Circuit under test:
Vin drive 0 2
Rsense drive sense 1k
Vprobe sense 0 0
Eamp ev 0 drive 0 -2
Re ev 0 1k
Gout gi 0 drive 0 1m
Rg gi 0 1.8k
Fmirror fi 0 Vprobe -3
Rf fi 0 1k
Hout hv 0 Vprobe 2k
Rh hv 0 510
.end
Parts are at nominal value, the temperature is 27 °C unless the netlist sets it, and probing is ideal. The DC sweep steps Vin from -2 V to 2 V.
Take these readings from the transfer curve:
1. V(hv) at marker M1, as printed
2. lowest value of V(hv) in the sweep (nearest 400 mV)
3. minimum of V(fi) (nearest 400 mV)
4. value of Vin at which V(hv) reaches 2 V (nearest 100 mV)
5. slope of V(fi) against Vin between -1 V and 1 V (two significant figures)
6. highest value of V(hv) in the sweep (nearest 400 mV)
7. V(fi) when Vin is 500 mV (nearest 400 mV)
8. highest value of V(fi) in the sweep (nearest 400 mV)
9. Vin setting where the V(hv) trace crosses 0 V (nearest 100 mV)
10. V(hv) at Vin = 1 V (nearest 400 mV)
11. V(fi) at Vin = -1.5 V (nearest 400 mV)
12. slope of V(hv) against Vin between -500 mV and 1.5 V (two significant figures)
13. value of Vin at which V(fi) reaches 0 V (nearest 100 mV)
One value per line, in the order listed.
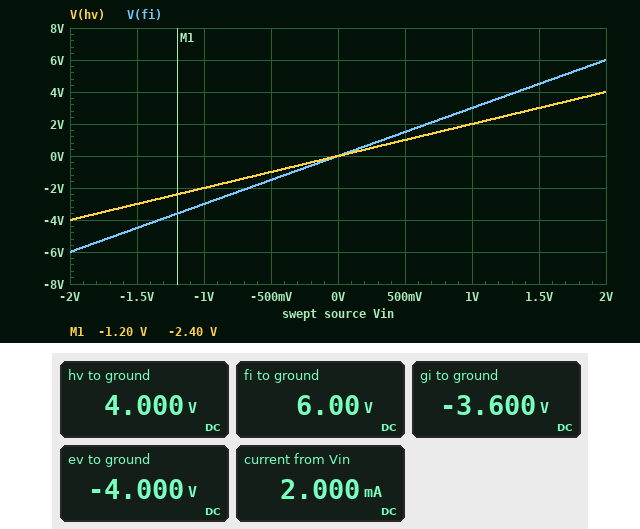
-2.40 V
-4.0 V
-6.0 V
1.0 V
3.0 V/V
4.0 V
1.6 V
6.0 V
0 V
2.0 V
-4.4 V
2.0 V/V
0 V
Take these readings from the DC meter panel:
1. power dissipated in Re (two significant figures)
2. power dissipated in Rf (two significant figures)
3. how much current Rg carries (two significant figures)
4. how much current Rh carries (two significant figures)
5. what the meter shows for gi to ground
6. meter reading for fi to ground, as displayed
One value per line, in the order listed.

16 mW
36 mW
2.0 mA
7.8 mA
-3.600 V
6.00 V
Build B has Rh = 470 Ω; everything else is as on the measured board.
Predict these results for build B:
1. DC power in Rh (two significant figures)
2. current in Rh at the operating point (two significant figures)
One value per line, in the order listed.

34 mW
8.5 mA
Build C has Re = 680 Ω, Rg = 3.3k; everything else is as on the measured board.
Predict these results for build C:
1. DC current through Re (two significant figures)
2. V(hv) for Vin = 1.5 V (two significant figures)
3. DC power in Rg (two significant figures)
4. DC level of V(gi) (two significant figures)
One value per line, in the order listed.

5.9 mA
3.0 V
13 mW
-6.6 V
